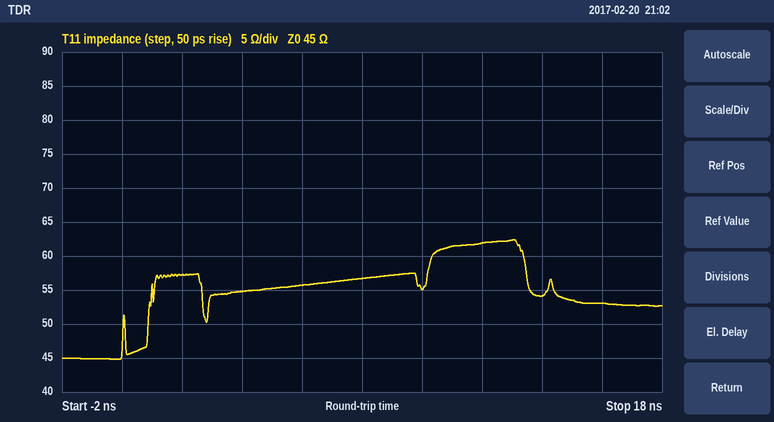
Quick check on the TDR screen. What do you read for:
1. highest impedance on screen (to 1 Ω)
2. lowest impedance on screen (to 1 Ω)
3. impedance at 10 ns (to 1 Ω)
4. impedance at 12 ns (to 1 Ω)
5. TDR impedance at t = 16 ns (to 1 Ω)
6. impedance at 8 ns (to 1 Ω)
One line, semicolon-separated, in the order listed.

62 Ω; 45 Ω; 55 Ω; 62 Ω; 53 Ω; 57 Ω
